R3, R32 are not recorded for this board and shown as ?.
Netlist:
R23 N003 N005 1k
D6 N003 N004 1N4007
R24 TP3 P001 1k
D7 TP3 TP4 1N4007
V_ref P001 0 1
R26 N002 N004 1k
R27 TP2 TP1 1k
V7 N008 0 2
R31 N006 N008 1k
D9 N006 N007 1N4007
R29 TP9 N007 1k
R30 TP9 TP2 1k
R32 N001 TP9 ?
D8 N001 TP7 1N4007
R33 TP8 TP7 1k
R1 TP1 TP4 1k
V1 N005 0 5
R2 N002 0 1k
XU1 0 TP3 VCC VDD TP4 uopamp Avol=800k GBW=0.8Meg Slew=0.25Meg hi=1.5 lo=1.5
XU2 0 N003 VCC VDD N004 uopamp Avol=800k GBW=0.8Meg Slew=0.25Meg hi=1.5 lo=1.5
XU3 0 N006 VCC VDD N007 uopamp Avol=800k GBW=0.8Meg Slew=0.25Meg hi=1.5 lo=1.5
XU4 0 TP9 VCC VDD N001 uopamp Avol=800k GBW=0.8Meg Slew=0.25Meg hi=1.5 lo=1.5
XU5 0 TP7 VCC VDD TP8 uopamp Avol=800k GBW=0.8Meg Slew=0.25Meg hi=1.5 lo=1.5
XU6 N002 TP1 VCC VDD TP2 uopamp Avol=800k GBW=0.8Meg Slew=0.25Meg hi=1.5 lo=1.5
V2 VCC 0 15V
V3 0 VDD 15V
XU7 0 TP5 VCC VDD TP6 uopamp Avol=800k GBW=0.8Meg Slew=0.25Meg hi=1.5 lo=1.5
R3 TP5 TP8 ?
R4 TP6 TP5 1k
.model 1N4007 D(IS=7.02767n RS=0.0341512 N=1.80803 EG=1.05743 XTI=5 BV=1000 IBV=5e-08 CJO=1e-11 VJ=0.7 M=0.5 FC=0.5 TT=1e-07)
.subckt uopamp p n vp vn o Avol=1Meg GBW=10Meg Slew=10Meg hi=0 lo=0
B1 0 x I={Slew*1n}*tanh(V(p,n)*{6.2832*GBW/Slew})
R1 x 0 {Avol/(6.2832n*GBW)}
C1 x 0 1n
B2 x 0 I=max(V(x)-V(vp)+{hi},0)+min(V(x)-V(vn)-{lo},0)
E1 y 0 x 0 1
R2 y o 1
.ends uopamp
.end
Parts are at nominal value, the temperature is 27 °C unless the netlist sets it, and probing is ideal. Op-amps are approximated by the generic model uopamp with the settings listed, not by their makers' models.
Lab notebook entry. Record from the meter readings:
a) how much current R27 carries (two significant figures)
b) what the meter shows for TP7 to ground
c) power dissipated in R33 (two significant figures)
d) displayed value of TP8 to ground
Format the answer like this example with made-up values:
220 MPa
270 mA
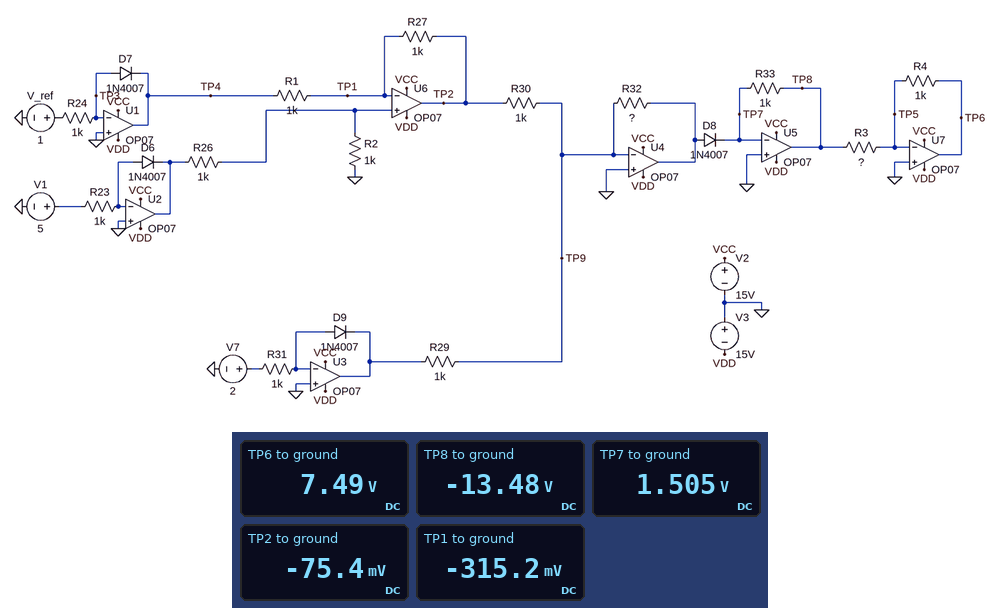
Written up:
240 µA
1.505 V
220 mW
-13.48 V
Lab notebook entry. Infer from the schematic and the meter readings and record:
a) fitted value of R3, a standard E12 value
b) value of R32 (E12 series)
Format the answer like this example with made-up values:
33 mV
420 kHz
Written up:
1.8 kΩ
3.3 kΩ
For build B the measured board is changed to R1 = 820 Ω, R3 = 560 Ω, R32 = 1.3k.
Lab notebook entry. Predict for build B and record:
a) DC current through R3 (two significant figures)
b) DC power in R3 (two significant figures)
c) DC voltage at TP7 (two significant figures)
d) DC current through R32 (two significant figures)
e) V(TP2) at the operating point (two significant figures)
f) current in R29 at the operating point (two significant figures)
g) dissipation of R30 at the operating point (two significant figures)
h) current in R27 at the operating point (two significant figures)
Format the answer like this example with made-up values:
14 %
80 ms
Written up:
17 mA
170 mW
120 mV
610 µA
-23 mV
590 µA
520 nW
290 µA
